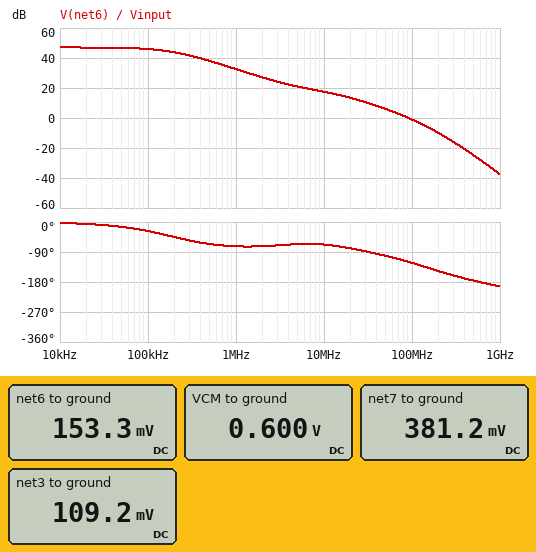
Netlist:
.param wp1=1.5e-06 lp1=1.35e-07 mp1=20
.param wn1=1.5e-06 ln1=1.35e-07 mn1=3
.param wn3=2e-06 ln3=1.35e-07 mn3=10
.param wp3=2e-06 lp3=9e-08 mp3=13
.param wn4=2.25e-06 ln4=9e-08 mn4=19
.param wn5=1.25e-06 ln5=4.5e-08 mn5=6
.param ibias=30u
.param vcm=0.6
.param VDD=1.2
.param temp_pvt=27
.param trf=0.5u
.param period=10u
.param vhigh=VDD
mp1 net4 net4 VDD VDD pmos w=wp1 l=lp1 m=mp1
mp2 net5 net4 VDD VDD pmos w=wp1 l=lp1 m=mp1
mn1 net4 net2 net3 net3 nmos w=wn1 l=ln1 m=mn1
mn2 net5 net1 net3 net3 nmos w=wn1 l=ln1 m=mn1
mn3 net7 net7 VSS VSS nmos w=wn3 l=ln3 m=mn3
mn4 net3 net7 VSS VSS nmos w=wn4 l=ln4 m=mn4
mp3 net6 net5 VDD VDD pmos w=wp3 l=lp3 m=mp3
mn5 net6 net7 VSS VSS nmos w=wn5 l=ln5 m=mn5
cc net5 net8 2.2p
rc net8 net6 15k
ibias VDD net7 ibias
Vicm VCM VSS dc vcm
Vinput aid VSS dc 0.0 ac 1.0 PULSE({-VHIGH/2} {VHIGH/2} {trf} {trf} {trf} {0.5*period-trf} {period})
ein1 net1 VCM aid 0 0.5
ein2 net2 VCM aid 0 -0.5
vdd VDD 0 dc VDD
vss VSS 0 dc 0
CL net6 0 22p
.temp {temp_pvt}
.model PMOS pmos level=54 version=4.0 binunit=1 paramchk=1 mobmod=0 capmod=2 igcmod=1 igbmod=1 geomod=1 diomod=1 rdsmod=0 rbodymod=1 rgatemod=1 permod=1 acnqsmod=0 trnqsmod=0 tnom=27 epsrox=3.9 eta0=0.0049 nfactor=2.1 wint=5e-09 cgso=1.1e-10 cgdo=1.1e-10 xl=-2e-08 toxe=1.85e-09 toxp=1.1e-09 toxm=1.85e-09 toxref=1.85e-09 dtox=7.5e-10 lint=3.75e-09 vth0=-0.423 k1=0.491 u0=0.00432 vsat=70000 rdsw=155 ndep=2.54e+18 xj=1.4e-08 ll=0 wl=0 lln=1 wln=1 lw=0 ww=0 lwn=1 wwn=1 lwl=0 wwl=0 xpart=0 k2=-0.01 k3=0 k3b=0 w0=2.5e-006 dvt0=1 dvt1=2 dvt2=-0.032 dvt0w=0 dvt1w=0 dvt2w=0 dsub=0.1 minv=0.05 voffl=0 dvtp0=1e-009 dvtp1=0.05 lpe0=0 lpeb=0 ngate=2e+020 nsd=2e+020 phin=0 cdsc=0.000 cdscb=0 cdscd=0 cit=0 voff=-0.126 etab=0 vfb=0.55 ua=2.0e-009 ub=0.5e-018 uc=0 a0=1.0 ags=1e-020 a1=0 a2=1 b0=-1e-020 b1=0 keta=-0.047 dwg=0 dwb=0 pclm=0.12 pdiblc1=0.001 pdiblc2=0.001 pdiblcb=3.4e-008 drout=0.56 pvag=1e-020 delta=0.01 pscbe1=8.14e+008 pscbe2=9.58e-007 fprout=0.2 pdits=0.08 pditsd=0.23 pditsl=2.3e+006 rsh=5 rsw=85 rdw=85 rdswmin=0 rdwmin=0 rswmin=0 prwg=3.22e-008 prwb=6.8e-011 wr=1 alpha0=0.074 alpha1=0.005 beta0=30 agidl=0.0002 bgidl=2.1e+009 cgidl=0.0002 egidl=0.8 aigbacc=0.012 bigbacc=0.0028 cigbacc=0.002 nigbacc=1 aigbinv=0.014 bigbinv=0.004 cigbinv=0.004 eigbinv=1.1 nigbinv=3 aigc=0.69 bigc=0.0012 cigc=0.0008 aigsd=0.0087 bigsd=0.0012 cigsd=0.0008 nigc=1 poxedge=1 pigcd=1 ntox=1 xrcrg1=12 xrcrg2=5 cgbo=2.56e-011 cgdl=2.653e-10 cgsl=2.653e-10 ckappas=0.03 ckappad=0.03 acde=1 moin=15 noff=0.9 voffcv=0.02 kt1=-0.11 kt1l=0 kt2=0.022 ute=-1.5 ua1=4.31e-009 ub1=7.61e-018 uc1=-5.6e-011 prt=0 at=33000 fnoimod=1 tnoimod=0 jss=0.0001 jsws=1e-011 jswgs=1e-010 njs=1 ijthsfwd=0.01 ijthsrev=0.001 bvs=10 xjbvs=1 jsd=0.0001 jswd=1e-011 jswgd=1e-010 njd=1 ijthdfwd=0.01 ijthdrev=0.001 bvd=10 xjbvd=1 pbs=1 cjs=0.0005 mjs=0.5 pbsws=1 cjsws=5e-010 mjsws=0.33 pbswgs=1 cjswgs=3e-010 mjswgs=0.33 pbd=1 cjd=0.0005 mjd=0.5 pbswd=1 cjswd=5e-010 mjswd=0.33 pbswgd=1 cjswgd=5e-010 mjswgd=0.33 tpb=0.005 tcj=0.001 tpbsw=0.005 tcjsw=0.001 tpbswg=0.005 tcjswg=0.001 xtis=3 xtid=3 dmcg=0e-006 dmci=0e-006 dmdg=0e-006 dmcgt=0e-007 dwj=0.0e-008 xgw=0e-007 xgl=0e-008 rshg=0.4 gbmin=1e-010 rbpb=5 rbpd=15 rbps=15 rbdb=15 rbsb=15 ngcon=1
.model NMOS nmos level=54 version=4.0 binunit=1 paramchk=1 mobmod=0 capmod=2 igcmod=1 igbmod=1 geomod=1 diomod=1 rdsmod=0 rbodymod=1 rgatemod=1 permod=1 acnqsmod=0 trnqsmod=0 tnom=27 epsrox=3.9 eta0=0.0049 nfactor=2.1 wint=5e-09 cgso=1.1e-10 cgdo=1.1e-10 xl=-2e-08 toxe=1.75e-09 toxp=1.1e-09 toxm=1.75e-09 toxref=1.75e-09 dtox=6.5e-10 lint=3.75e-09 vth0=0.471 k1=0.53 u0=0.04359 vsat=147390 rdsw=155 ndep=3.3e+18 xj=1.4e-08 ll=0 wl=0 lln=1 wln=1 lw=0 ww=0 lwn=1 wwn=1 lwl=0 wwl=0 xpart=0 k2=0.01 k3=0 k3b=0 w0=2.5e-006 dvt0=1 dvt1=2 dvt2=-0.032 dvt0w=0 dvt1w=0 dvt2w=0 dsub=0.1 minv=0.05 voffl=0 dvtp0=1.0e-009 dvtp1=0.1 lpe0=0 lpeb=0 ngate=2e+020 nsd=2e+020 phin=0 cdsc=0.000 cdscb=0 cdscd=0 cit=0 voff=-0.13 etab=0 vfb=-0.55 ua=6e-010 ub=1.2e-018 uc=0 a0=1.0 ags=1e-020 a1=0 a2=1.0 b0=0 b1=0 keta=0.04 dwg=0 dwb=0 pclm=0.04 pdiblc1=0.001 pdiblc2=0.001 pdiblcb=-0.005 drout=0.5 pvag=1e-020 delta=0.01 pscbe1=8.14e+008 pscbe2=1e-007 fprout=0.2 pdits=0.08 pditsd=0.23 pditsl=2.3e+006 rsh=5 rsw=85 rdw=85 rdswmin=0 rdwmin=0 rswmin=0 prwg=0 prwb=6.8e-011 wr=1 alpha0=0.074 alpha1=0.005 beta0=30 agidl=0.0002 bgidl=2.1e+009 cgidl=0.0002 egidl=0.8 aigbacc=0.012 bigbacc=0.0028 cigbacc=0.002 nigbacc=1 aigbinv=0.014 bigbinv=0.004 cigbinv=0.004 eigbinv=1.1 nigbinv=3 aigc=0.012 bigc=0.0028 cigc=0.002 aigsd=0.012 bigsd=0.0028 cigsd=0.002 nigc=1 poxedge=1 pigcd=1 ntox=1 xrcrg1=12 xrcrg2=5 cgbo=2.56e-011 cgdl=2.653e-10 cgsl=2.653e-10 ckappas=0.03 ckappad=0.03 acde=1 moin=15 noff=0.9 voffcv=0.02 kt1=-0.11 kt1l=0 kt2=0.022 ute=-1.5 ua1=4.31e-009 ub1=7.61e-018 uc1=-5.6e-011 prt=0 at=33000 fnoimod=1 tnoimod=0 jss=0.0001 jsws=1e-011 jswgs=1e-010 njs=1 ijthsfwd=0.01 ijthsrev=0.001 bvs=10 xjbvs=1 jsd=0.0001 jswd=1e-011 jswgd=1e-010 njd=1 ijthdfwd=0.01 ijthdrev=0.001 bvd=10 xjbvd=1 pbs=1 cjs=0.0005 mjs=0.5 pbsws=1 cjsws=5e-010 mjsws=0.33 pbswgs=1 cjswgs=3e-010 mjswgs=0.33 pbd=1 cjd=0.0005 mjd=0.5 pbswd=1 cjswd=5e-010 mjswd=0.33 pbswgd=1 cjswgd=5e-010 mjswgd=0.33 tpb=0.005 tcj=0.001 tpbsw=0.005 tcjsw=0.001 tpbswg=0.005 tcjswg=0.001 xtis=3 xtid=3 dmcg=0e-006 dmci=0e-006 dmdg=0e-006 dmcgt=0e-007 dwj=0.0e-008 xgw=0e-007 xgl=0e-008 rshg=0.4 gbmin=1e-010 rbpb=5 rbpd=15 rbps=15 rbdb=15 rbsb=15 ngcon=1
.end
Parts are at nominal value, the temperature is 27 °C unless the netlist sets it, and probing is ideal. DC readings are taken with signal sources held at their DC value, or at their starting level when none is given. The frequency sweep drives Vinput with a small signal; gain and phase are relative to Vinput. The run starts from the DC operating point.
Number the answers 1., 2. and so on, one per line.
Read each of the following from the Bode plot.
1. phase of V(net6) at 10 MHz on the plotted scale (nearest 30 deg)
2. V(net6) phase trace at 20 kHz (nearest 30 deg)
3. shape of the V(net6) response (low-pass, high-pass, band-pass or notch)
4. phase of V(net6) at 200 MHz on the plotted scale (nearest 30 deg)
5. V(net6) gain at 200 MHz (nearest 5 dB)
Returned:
1. -60 deg
2. 0 deg
3. low-pass
4. -150 deg
5. -10 dB
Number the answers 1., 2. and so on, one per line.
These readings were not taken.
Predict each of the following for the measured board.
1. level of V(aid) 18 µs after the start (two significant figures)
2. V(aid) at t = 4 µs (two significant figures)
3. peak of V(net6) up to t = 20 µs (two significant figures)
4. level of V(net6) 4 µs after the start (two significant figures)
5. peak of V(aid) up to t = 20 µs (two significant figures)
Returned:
1. -600 mV
2. 600 mV
3. 1.1 V
4. 1.1 V
5. 600 mV
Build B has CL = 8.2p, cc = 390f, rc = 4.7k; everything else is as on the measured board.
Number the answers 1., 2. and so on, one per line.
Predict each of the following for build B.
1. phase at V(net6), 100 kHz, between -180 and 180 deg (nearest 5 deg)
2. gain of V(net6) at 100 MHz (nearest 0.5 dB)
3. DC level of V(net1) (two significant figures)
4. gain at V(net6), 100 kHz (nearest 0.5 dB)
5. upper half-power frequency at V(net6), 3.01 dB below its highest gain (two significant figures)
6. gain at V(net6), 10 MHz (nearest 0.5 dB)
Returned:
1. -5 deg
2. 0.5 dB
3. 600 mV
4. 47.0 dB
5. 1.0 MHz
6. 26.5 dB
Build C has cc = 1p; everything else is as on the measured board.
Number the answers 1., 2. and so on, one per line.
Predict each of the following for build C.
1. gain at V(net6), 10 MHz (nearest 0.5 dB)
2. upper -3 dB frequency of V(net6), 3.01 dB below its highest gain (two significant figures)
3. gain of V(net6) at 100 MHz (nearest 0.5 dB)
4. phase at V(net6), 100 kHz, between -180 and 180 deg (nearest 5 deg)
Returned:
1. 19.5 dB
2. 390 kHz
3. -1.0 dB
4. -15 deg
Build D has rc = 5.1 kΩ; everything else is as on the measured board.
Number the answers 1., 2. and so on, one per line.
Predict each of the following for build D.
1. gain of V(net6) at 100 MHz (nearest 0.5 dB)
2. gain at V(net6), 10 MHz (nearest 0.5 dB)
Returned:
1. -9.0 dB
2. 12.5 dB
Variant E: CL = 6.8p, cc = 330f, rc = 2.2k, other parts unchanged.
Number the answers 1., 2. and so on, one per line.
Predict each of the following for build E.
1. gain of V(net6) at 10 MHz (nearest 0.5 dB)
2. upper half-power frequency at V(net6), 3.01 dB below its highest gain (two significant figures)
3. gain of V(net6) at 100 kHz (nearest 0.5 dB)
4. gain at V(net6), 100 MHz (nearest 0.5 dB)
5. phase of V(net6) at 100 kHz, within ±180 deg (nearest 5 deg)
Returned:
1. 28.0 dB
2. 1.2 MHz
3. 47.0 dB
4. 0.5 dB
5. -5 deg
